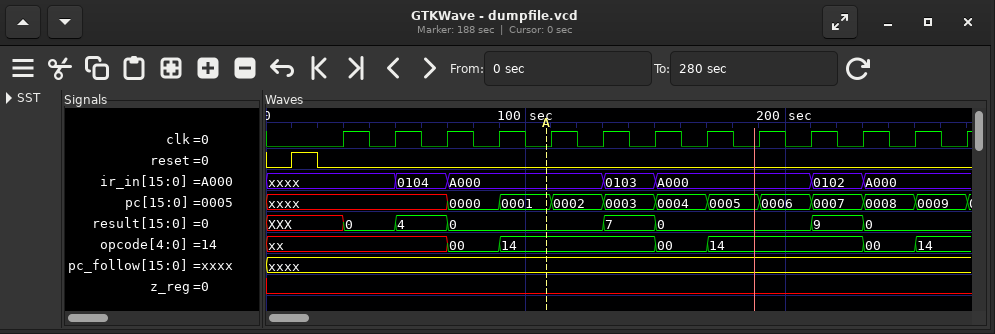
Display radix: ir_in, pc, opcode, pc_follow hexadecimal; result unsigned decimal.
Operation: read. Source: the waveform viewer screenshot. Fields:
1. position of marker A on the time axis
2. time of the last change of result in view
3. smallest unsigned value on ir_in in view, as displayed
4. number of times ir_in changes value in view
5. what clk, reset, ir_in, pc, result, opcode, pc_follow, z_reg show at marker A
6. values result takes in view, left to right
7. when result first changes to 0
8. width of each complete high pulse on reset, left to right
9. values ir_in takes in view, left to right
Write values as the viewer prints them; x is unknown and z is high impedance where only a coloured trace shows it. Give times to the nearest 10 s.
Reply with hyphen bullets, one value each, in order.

- 110 s
- 230 s
- 0102
- 6
- clk=0, reset=0, ir_in=A000, pc=0001, result=0, opcode=14, pc_follow=xxxx, z_reg=0
- XXX, 0, 4, 0, 7, 0, 9, 0
- 30 s
- 10 s
- xxxx, 0104, A000, 0103, A000, 0102, A000
